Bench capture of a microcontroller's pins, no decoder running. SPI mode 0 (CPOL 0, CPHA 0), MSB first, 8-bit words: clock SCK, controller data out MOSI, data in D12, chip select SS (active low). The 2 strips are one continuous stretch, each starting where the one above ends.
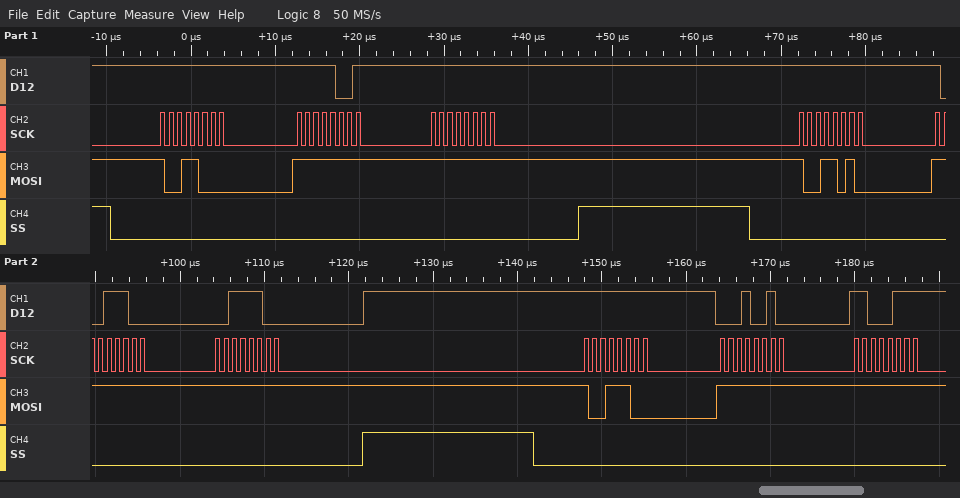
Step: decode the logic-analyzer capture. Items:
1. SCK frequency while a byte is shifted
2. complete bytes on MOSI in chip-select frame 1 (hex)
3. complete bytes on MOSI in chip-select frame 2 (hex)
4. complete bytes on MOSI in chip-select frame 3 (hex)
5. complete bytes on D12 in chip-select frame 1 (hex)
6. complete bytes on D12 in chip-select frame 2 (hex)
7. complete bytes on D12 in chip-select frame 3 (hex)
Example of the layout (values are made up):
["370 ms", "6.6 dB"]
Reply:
["1 MHz", "0x98 0xFF 0xFF", "0x9A 0xFF 0xFF", "0x9C 0xFF 0xFF", "0xFF 0xF9 0xFF", "0xFF 0x9C 0x3C", "0xFF 0x12 0xC7"]
